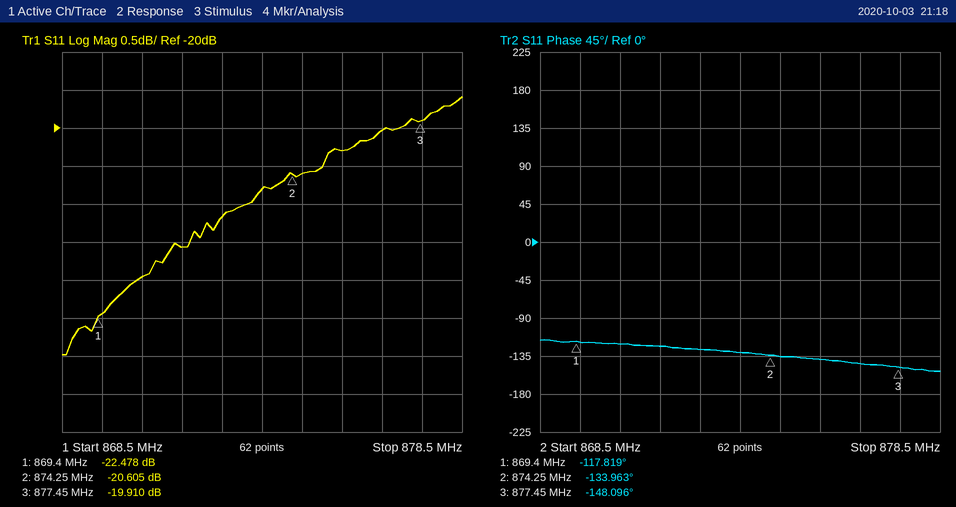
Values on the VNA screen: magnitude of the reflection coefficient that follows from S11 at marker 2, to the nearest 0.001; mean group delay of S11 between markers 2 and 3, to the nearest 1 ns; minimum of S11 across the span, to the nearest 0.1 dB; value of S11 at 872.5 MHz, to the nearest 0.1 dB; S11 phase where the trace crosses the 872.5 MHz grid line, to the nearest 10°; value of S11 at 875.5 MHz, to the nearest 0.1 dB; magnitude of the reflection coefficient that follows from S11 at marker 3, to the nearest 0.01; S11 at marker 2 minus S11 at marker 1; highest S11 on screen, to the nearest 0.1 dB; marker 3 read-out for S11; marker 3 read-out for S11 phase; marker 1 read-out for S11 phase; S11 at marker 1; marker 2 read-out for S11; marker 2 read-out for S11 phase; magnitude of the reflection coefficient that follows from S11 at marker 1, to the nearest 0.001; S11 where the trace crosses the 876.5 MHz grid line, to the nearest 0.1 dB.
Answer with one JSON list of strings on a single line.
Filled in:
["0.093", "12 ns", "-23.0 dB", "-21.2 dB", "-130°", "-20.3 dB", "0.10", "1.873 dB", "-19.6 dB", "-19.910 dB", "-148.096°", "-117.819°", "-22.478 dB", "-20.605 dB", "-133.963°", "0.075", "-20.0 dB"]
